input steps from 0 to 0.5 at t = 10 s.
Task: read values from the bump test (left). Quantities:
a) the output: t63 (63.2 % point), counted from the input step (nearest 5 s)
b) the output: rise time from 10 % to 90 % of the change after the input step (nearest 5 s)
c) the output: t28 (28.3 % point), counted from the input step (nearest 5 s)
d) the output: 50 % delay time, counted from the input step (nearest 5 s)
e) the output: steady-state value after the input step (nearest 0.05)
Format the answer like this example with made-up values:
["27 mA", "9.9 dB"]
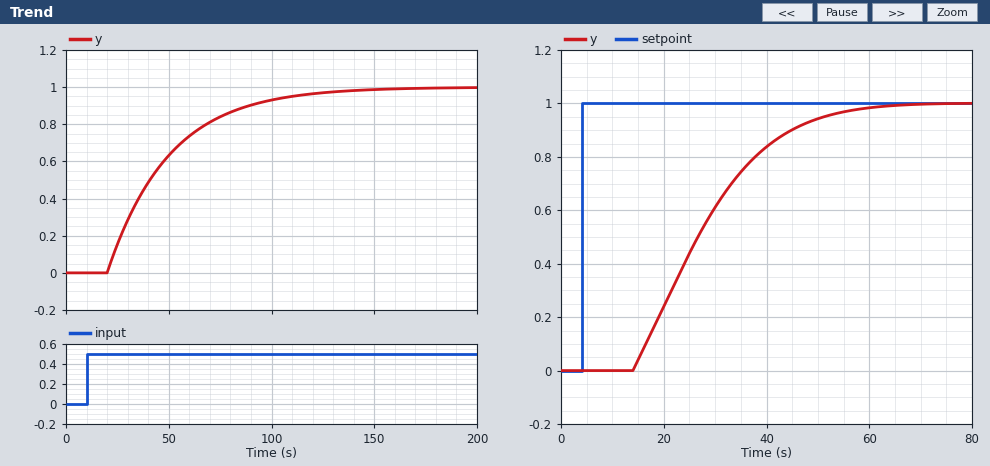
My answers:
["40 s", "65 s", "20 s", "30 s", "1.00"]
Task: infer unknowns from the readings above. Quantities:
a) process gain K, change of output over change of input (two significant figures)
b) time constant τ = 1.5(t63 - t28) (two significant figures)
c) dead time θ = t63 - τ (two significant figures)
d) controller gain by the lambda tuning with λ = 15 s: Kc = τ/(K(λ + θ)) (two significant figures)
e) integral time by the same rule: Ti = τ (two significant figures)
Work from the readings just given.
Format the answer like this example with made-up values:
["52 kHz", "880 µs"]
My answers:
["2.0", "30 s", "10 s", "0.60", "30 s"]
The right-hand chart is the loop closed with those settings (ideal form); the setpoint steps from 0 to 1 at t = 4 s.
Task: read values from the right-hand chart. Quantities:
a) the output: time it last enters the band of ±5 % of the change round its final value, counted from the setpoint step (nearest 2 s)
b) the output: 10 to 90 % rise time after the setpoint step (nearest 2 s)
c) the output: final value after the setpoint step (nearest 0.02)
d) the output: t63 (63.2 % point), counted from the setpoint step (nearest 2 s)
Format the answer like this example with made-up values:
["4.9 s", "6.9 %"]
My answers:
["48 s", "28 s", "1.00", "26 s"]
